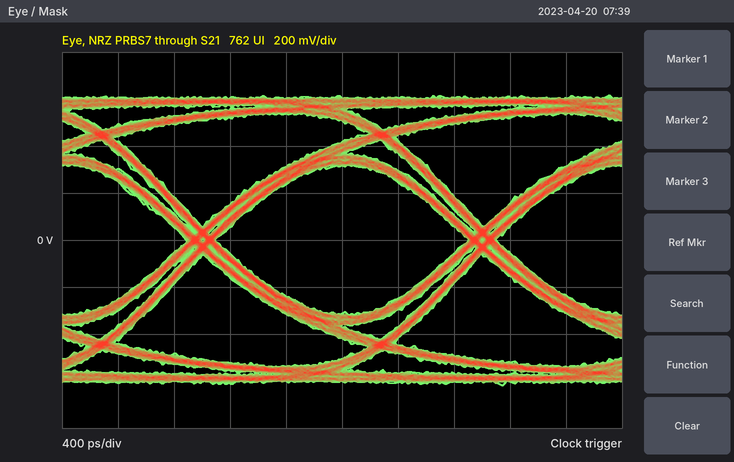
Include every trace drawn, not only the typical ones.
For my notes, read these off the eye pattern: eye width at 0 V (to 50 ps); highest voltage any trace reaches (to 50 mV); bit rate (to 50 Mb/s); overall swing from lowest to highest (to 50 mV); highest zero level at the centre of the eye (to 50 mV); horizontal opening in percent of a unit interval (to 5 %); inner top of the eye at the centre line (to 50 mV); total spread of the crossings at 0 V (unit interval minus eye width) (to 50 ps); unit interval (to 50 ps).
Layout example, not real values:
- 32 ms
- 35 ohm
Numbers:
- 1.80 ns
- 600 mV
- 500 Mb/s
- 1.25 V
- -300 mV
- 90 %
- 300 mV
- 200 ps
- 2.00 ns
